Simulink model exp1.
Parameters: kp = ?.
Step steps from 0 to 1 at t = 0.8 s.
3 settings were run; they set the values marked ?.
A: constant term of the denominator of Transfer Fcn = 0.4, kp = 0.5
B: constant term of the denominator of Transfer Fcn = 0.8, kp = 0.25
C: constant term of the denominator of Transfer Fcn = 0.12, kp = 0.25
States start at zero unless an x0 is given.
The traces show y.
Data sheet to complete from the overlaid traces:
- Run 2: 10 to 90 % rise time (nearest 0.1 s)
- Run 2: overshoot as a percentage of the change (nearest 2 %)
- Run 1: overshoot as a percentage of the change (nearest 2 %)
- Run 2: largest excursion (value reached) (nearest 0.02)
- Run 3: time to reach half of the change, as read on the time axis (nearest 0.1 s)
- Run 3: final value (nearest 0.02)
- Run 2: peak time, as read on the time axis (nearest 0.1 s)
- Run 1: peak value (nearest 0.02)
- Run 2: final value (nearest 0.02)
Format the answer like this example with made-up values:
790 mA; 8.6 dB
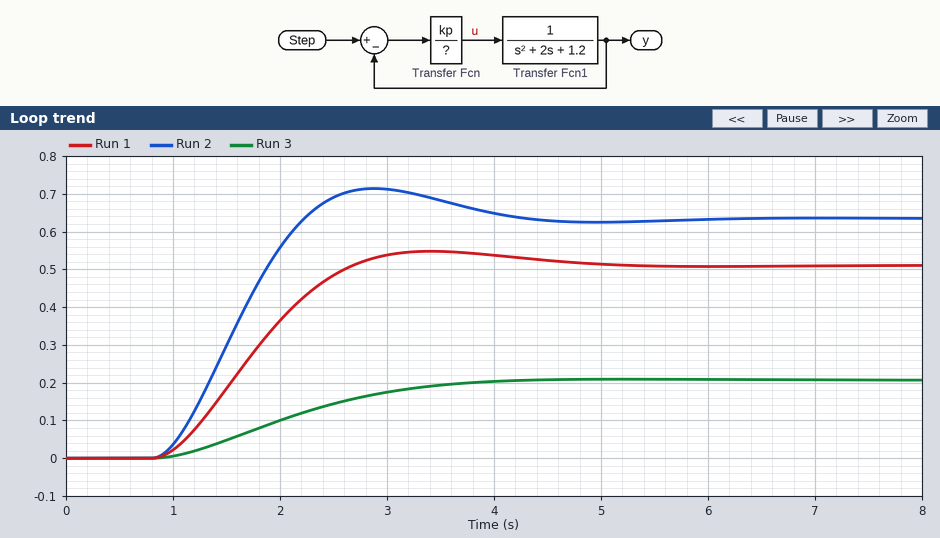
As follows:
1.0 s; 12 %; 8 %; 0.72; 2.0 s; 0.20; 2.9 s; 0.54; 0.64
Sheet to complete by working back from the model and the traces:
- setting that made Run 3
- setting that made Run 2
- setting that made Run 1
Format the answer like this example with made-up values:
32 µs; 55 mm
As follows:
B; C; A
